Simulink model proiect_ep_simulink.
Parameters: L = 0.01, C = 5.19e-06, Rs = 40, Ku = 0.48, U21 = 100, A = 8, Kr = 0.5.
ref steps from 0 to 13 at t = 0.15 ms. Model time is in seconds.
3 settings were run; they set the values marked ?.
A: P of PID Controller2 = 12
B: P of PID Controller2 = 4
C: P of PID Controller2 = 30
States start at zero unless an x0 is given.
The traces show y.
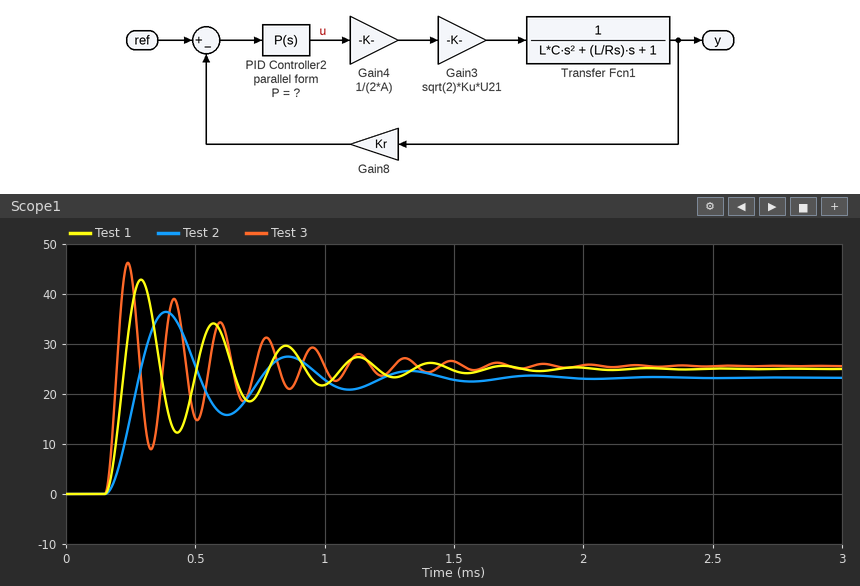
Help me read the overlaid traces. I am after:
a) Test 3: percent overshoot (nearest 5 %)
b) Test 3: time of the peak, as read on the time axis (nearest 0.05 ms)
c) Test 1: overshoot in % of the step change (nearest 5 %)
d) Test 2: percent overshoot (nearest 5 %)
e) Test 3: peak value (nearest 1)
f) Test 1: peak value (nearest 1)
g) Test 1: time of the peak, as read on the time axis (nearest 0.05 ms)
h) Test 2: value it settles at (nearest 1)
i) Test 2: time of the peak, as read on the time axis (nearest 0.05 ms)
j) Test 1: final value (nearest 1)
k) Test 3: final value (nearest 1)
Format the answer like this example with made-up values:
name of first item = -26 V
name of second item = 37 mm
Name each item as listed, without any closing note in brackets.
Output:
Test 3: percent overshoot = 80 %
Test 3: time of the peak, as read on the time axis = 0.25 ms
Test 1: overshoot in % of the step change = 70 %
Test 2: percent overshoot = 55 %
Test 3: peak value = 46
Test 1: peak value = 43
Test 1: time of the peak, as read on the time axis = 0.30 ms
Test 2: value it settles at = 23
Test 2: time of the peak, as read on the time axis = 0.40 ms
Test 1: final value = 25
Test 3: final value = 26
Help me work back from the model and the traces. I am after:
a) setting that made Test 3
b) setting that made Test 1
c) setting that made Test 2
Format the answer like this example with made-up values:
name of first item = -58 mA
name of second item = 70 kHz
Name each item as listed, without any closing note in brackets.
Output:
setting that made Test 3 = C
setting that made Test 1 = A
setting that made Test 2 = B
